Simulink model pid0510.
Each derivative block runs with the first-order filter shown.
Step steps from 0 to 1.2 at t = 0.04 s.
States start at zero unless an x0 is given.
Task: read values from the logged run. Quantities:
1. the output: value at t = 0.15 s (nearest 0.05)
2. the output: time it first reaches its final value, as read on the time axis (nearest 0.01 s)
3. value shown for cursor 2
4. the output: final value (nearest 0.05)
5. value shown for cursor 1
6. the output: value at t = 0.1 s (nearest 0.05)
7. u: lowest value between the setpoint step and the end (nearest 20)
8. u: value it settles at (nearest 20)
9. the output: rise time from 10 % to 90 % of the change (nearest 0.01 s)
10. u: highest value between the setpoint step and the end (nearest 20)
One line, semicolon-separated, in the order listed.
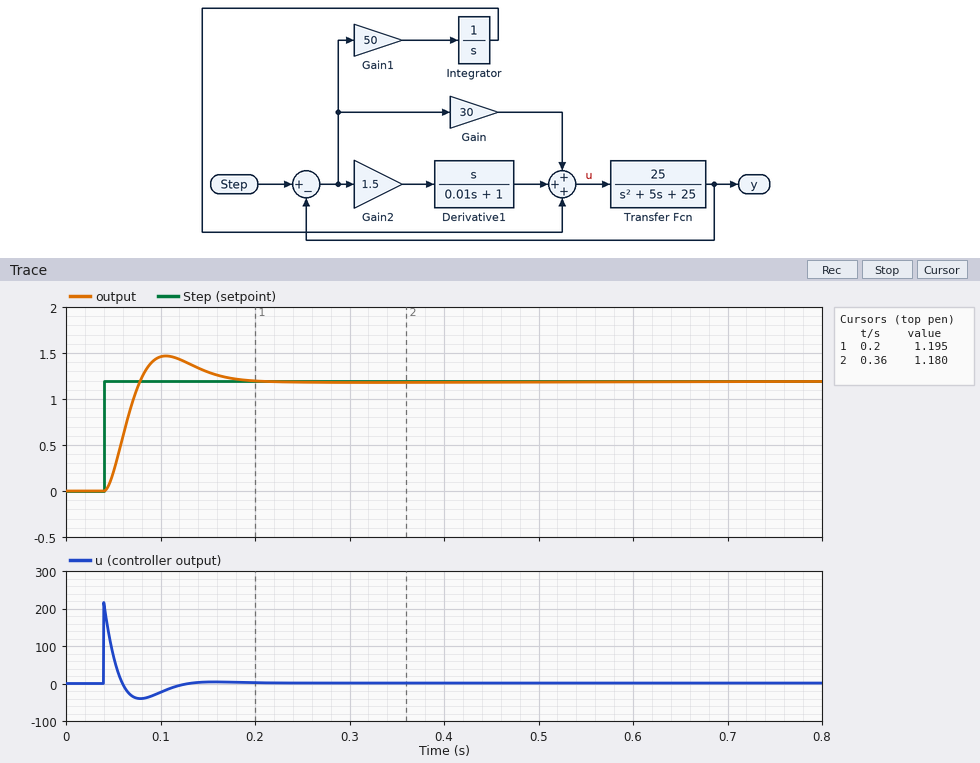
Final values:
1.30; 0.08 s; 1.180; 1.20; 1.195; 1.45; -40; 0; 0.03 s; 220
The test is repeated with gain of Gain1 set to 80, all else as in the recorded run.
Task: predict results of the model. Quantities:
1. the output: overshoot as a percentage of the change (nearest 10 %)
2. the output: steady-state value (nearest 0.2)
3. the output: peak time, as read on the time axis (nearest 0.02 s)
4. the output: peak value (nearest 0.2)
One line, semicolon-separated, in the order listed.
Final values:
20 %; 1.2; 0.10 s; 1.4
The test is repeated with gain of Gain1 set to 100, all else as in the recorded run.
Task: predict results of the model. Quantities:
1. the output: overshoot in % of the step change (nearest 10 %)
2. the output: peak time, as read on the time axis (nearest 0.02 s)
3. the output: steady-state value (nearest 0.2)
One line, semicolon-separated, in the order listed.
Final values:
20 %; 0.10 s; 1.2
